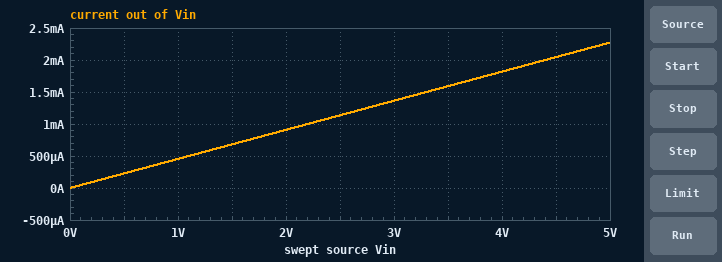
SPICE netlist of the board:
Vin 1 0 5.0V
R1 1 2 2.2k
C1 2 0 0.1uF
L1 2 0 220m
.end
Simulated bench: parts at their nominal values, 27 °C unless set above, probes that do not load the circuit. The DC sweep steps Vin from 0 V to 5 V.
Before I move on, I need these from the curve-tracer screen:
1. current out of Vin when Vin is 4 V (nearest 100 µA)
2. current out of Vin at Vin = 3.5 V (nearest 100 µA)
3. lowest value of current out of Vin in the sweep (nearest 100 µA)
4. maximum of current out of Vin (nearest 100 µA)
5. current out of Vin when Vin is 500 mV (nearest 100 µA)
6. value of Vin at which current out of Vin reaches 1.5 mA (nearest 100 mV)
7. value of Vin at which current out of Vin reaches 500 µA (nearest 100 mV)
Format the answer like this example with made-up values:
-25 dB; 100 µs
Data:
1.8 mA; 1.6 mA; 0 A; 2.3 mA; 200 µA; 3.3 V; 1.1 V
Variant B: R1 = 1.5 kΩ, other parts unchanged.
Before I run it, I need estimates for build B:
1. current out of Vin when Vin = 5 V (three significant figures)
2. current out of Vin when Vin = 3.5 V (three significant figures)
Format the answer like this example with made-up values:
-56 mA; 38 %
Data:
3.33 mA; 2.33 mA
